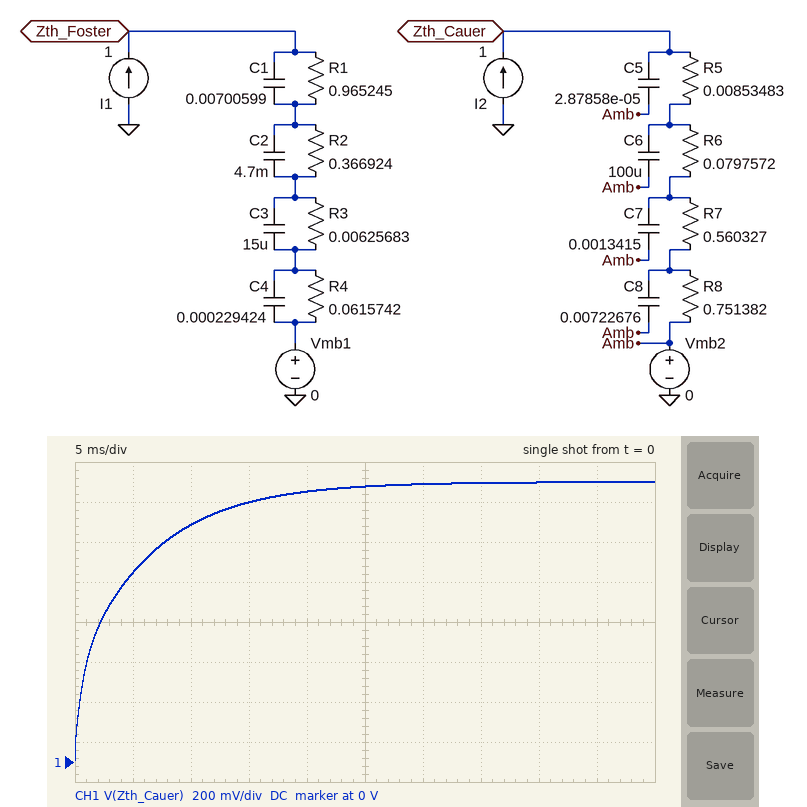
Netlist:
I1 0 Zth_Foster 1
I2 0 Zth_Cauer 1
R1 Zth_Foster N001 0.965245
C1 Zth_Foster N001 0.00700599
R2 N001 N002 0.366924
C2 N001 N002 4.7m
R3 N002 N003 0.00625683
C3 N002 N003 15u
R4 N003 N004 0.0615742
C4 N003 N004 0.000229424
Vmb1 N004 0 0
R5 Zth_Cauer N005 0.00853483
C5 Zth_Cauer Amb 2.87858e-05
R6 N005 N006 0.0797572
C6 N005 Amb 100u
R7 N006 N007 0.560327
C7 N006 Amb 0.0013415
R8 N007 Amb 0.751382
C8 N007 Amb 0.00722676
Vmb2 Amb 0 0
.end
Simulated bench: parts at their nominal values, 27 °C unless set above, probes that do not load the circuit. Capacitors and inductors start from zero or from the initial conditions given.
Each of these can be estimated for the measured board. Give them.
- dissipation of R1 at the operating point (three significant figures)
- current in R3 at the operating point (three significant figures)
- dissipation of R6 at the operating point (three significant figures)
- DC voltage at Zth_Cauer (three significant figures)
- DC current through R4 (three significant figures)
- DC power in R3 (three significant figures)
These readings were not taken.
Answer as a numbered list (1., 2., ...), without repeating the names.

1. 965 mW
2. 1.00 A
3. 79.8 mW
4. 1.40 V
5. 1.00 A
6. 6.26 mW
